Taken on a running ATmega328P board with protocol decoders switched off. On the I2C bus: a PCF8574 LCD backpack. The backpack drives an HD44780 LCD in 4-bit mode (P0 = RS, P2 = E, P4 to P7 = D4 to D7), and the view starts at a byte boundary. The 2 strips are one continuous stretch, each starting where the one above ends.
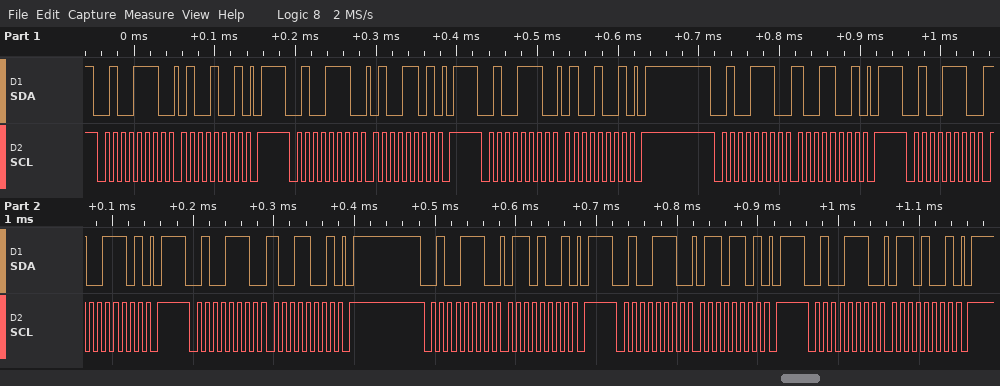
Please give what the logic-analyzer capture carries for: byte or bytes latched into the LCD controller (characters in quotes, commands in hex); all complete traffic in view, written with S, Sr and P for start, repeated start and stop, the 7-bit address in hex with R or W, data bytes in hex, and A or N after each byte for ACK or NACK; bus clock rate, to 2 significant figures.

'I'
S 27W A 49 A P S 27W A 4D A P S 27W A 49 A P S 27W A 99 A P S 27W A 9D A P S 27W A 99 A P S 27W A 69 A P S 27W A 6D A P S 27W A 69 A P
100 kHz
